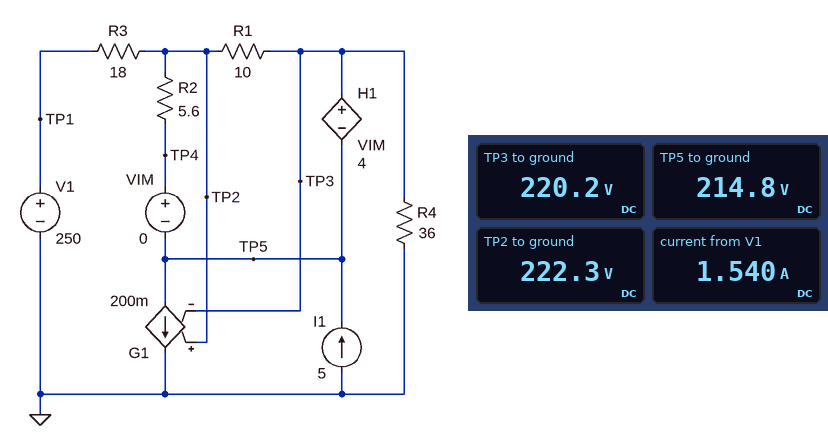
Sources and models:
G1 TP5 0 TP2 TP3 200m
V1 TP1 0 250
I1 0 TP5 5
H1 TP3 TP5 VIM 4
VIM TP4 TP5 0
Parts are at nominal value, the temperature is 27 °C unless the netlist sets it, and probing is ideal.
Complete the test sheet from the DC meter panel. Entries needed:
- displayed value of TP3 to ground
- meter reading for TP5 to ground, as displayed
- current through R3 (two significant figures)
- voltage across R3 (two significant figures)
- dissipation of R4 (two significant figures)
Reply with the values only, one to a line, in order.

220.2 V
214.8 V
1.5 A
28 V
1.3 kW
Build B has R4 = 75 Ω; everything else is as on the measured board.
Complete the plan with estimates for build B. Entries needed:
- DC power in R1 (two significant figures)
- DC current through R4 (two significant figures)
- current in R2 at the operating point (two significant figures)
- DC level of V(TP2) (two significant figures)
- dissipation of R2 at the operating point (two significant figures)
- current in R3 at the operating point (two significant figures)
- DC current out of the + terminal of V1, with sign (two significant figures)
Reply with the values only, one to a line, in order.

550 mW
3.8 A
1.5 A
280 V
12 W
1.7 A
-1.7 A
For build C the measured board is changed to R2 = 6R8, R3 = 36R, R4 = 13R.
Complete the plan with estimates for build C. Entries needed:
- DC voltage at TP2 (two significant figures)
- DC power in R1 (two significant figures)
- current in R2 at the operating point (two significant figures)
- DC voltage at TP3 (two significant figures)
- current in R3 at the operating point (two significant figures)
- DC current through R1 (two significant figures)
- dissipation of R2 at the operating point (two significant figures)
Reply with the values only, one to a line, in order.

100 V
7.9 W
3.2 A
95 V
4.1 A
890 mA
69 W
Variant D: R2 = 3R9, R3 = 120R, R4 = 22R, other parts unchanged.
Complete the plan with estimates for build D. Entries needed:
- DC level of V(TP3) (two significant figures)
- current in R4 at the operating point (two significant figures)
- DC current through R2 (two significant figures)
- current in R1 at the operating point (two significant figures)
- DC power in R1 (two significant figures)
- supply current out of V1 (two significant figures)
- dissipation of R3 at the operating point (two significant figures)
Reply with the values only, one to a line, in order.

130 V
6.0 A
990 mA
9.9 mA
990 µW
980 mA
120 W
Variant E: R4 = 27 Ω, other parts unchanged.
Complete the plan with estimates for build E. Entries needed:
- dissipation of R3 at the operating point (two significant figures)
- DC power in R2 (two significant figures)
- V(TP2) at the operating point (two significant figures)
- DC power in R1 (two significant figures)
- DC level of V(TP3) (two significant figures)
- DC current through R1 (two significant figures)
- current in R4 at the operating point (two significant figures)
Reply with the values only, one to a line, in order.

160 W
36 W
200 V
1.7 W
190 V
410 mA
7.1 A
